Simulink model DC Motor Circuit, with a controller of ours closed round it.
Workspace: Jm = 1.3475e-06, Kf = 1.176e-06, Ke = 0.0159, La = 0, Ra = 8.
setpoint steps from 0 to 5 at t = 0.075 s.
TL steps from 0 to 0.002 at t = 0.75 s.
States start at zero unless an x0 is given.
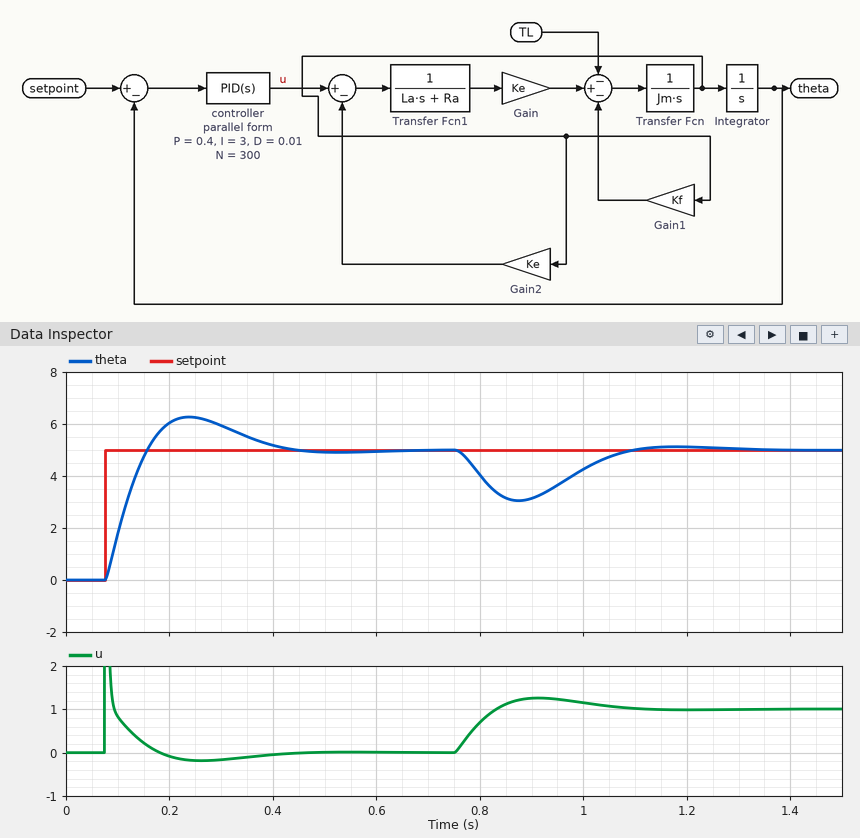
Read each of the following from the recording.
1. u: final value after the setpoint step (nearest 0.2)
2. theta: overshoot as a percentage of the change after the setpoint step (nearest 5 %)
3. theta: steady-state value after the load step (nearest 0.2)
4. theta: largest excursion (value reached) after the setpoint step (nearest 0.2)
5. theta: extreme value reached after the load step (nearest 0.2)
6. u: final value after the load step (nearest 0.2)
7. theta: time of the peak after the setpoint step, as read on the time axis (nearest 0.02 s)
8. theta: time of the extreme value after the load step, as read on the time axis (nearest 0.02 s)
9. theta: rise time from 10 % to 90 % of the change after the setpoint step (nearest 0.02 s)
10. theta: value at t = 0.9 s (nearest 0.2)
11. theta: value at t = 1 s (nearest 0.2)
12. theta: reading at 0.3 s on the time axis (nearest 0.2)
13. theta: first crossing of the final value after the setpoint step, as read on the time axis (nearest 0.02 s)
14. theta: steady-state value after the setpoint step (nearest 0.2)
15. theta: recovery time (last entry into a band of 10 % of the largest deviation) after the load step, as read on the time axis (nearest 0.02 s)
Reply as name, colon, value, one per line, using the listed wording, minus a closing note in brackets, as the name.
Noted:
u: final value after the setpoint step: 0.0
theta: overshoot as a percentage of the change after the setpoint step: 25 %
theta: steady-state value after the load step: 5.0
theta: largest excursion (value reached) after the setpoint step: 6.2
theta: extreme value reached after the load step: 3.0
u: final value after the load step: 1.0
theta: time of the peak after the setpoint step, as read on the time axis: 0.24 s
theta: time of the extreme value after the load step, as read on the time axis: 0.88 s
theta: rise time from 10 % to 90 % of the change after the setpoint step: 0.06 s
theta: value at t = 0.9 s: 3.2
theta: value at t = 1 s: 4.2
theta: reading at 0.3 s on the time axis: 6.0
theta: first crossing of the final value after the setpoint step, as read on the time axis: 0.16 s
theta: steady-state value after the setpoint step: 5.0
theta: recovery time (last entry into a band of 10 % of the largest deviation) after the load step, as read on the time axis: 1.06 s
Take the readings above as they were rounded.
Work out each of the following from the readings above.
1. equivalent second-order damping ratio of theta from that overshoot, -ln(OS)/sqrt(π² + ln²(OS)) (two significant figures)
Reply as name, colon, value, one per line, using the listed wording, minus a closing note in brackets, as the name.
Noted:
equivalent second-order damping ratio of theta from that overshoot, -ln(OS)/sqrt(π² + ln²(OS)): 0.40
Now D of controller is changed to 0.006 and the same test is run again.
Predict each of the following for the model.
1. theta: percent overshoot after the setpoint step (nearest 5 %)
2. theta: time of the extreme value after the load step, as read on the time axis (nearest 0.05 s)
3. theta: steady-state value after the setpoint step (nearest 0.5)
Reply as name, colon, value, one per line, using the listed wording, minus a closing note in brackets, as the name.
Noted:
theta: percent overshoot after the setpoint step: 35 %
theta: time of the extreme value after the load step, as read on the time axis: 0.85 s
theta: steady-state value after the setpoint step: 5.0
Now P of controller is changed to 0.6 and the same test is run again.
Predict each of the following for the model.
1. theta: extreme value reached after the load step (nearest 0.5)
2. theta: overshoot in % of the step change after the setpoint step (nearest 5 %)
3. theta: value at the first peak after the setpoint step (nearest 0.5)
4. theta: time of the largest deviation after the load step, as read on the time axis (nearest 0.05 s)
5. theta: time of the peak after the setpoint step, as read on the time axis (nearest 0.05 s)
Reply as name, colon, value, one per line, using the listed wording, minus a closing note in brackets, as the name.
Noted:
theta: extreme value reached after the load step: 3.5
theta: overshoot in % of the step change after the setpoint step: 20 %
theta: value at the first peak after the setpoint step: 6.0
theta: time of the largest deviation after the load step, as read on the time axis: 0.85 s
theta: time of the peak after the setpoint step, as read on the time axis: 0.20 s
